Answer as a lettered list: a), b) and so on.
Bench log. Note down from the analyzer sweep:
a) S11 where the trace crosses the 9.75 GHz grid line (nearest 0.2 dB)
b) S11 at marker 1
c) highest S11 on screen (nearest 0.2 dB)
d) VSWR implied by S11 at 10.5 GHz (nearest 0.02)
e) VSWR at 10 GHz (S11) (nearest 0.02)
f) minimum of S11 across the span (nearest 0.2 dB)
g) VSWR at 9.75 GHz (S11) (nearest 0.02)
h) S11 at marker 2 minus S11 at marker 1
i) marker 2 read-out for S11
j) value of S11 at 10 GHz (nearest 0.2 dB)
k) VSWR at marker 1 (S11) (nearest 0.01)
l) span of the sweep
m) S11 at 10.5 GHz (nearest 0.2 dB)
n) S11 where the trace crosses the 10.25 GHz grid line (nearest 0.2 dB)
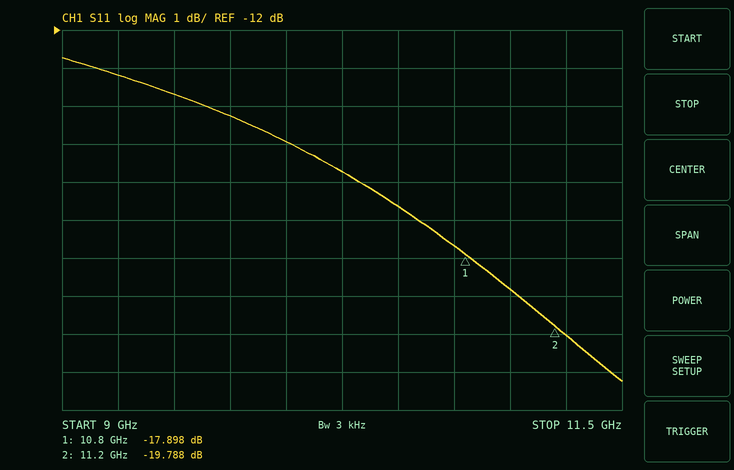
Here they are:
a) -14.2 dB
b) -17.898 dB
c) -12.8 dB
d) 1.34
e) 1.44
f) -21.2 dB
g) 1.48
h) -1.890 dB
i) -19.788 dB
j) -15.0 dB
k) 1.29
l) 2.5 GHz
m) -16.6 dB
n) -15.8 dB
